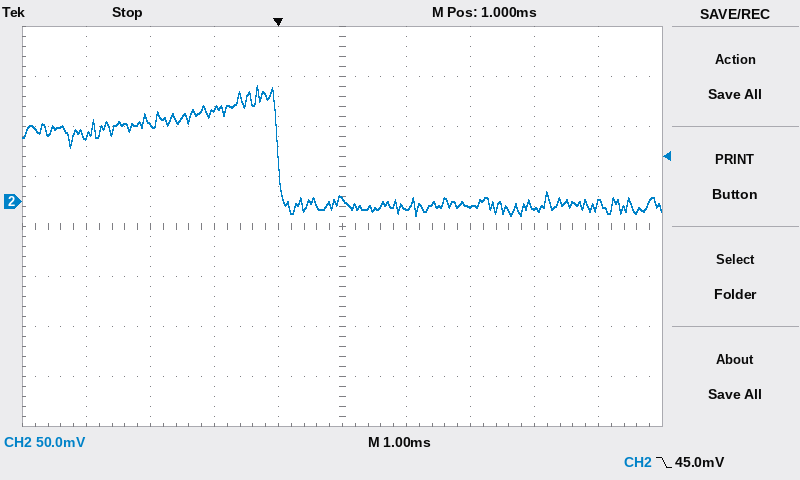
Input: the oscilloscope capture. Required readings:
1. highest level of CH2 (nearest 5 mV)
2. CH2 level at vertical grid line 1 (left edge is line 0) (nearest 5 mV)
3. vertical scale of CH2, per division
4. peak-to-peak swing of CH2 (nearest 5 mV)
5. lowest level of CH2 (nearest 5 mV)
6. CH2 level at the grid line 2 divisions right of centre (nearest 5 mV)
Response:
115 mV
65 mV
50 mV
130 mV
-15 mV
-5 mV
